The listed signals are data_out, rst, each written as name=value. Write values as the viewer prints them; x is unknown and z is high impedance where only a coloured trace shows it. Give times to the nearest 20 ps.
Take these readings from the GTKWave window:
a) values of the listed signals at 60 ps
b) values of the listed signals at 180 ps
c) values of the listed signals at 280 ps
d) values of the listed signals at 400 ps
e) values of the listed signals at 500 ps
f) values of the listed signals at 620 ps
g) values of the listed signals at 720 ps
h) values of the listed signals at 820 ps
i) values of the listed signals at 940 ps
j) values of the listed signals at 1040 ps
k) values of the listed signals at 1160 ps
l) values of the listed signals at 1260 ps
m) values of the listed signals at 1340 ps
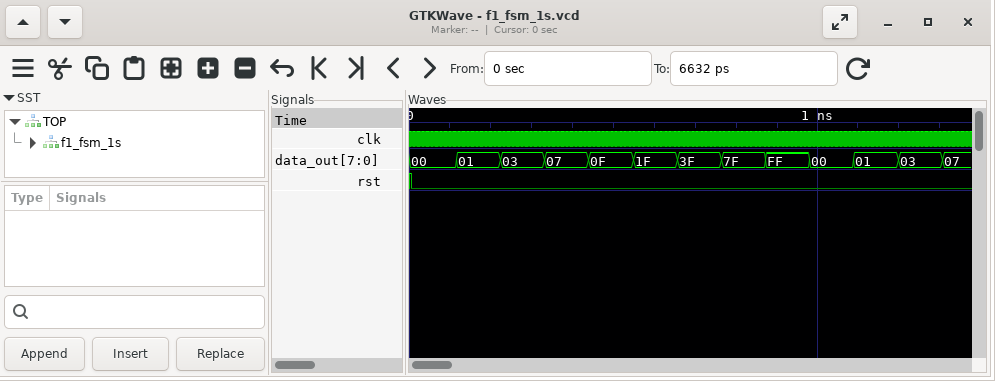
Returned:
data_out=00, rst=0
data_out=01, rst=0
data_out=03, rst=0
data_out=07, rst=0
data_out=0F, rst=0
data_out=1F, rst=0
data_out=3F, rst=0
data_out=7F, rst=0
data_out=FF, rst=0
data_out=00, rst=0
data_out=01, rst=0
data_out=03, rst=0
data_out=07, rst=0
